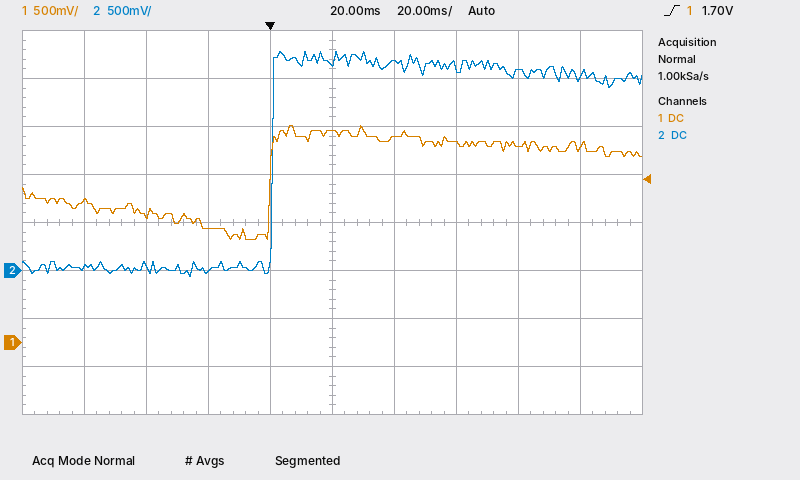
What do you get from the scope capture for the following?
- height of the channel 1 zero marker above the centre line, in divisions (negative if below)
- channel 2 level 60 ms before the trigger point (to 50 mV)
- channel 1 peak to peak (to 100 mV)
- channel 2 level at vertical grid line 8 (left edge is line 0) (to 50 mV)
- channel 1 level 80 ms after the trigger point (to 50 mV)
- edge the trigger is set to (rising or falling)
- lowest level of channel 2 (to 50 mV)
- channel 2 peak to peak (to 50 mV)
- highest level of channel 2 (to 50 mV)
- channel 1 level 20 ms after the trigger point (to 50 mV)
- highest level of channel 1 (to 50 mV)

-2.5 div
50 mV
1.20 V
2.10 V
2.05 V
rising
-50 mV
2.35 V
2.30 V
2.20 V
2.25 V
